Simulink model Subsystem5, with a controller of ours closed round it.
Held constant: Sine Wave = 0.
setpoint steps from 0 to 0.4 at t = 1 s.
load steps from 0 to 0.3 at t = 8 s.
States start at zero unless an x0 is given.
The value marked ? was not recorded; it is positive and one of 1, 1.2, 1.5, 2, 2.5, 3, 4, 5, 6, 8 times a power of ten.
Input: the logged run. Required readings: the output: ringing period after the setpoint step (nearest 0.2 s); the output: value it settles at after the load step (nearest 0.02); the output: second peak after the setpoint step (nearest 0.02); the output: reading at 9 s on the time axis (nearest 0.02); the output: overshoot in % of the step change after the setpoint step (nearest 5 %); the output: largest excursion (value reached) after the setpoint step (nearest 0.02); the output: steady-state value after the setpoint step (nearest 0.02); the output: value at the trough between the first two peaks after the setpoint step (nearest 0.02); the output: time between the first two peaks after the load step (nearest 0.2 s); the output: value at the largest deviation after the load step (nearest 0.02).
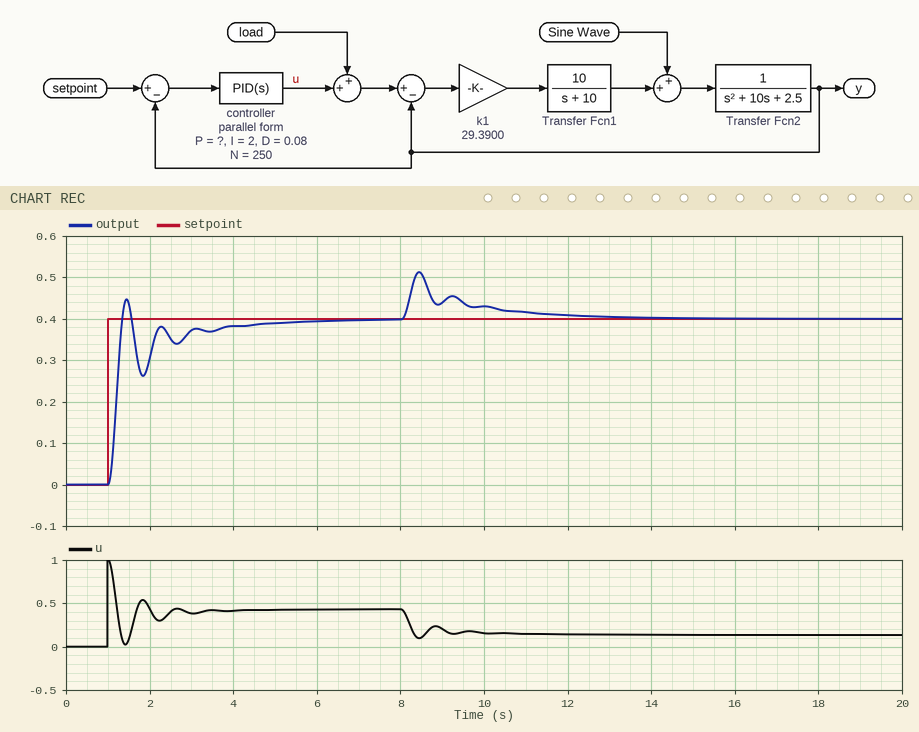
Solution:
0.8 s
0.40
0.38
0.44
10 %
0.44
0.40
0.26
0.8 s
0.52
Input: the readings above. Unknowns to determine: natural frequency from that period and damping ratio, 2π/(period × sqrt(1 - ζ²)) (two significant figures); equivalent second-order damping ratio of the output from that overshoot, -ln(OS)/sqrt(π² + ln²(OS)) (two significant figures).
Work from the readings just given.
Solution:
9.7 rad/s
0.59
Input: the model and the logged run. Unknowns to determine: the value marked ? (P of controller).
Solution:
2.5
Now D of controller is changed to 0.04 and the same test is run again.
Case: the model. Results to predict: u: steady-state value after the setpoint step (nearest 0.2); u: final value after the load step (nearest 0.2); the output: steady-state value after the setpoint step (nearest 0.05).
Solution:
0.4
0.2
0.40
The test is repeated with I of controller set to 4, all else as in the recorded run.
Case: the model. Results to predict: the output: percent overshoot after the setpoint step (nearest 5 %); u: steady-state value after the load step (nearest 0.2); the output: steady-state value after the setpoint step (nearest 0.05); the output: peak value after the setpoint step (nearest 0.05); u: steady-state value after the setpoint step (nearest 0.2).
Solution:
25 %
0.2
0.40
0.50
0.4
